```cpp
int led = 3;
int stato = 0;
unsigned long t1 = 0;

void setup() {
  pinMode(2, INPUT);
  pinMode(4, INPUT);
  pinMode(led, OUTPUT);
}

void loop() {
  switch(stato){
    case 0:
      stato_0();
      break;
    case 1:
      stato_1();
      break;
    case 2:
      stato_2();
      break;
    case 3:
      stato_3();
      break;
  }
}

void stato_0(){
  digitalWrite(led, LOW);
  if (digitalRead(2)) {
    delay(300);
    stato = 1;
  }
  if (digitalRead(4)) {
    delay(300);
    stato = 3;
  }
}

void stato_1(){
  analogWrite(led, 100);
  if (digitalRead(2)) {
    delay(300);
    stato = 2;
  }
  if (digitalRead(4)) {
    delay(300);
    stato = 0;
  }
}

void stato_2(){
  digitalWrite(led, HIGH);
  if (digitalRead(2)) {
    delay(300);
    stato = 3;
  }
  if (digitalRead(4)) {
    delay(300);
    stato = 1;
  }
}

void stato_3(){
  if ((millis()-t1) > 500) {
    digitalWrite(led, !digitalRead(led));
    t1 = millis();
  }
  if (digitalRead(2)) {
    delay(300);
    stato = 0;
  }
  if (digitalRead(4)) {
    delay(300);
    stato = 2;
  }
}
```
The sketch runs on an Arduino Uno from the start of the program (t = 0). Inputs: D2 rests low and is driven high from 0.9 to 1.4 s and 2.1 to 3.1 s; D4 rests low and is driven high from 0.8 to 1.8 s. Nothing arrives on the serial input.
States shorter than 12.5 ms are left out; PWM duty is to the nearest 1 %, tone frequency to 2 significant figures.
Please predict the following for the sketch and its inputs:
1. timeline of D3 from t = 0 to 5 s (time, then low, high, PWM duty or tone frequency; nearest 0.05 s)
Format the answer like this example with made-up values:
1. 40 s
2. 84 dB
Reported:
1. 0 s low; 1.1 s high; 2 s PWM 39 %; 2.4 s high; 2.7 s low; 3.3 s PWM 39 %
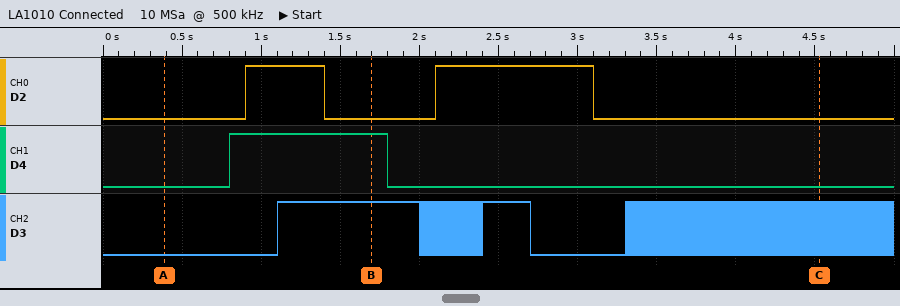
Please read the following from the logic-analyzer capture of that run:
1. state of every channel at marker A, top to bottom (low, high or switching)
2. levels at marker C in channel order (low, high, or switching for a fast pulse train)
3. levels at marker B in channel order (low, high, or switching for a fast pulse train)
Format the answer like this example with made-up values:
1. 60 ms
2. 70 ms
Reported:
1. D2 low, D4 low, D3 low
2. D2 low, D4 low, D3 switching
3. D2 low, D4 high, D3 high
